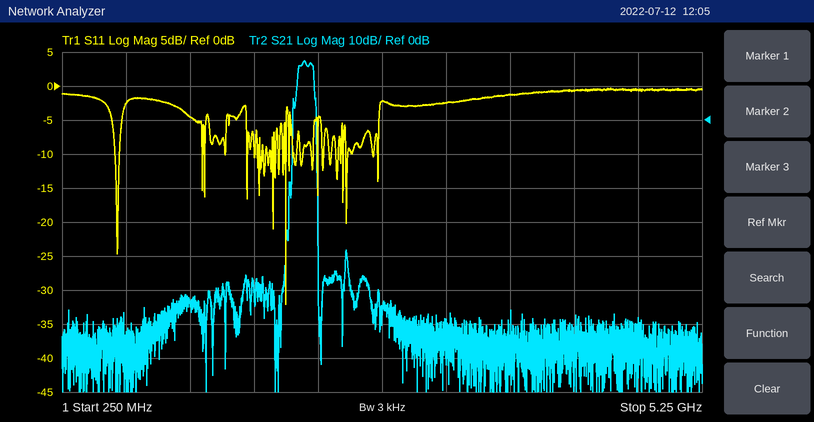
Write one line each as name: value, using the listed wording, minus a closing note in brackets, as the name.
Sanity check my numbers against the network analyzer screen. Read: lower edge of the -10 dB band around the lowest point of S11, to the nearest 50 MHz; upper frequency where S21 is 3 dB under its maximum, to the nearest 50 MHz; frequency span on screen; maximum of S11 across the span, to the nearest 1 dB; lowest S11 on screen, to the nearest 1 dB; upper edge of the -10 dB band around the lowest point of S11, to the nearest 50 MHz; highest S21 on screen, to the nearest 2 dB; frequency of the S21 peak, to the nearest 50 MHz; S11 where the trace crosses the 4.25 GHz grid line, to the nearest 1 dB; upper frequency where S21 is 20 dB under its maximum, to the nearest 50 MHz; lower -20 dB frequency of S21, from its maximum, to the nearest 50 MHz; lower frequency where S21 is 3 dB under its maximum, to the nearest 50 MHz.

lower edge of the -10 dB band around the lowest point of S11, to the nearest 50 MHz: 2.00 GHz
upper frequency where S21 is 3 dB under its maximum, to the nearest 50 MHz: 2.20 GHz
frequency span on screen: 5 GHz
maximum of S11 across the span, to the nearest 1 dB: 0 dB
lowest S11 on screen, to the nearest 1 dB: -32 dB
upper edge of the -10 dB band around the lowest point of S11, to the nearest 50 MHz: 2.00 GHz
highest S21 on screen, to the nearest 2 dB: 18 dB
frequency of the S21 peak, to the nearest 50 MHz: 2.15 GHz
S11 where the trace crosses the 4.25 GHz grid line, to the nearest 1 dB: -1 dB
upper frequency where S21 is 20 dB under its maximum, to the nearest 50 MHz: 2.25 GHz
lower -20 dB frequency of S21, from its maximum, to the nearest 50 MHz: 2.05 GHz
lower frequency where S21 is 3 dB under its maximum, to the nearest 50 MHz: 2.10 GHz
